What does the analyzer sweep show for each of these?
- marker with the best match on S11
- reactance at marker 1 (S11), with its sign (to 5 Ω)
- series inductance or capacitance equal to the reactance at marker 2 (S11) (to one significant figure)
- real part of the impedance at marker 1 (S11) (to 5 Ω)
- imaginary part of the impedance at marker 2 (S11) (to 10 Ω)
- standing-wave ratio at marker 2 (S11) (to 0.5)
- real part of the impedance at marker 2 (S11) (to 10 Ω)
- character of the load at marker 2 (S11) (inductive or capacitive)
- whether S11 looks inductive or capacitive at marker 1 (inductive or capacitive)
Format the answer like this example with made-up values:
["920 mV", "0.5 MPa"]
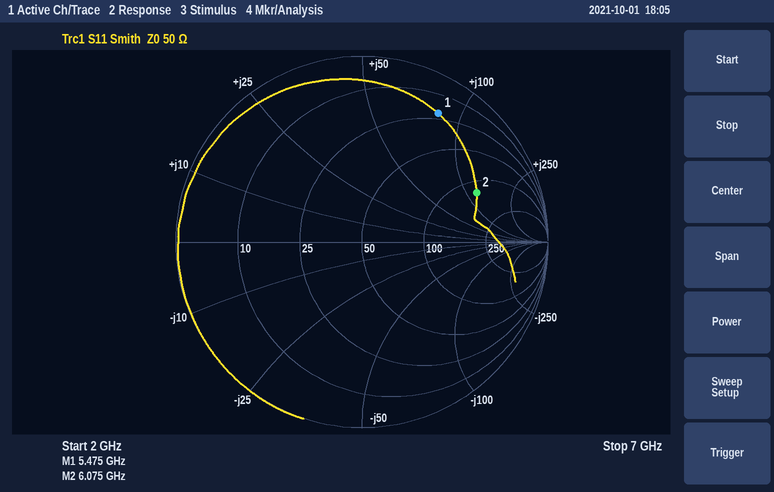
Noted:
["marker 2", "+85 Ω", "3 nH", "20 Ω", "+120 Ω", "5.0", "130 Ω", "inductive", "inductive"]
